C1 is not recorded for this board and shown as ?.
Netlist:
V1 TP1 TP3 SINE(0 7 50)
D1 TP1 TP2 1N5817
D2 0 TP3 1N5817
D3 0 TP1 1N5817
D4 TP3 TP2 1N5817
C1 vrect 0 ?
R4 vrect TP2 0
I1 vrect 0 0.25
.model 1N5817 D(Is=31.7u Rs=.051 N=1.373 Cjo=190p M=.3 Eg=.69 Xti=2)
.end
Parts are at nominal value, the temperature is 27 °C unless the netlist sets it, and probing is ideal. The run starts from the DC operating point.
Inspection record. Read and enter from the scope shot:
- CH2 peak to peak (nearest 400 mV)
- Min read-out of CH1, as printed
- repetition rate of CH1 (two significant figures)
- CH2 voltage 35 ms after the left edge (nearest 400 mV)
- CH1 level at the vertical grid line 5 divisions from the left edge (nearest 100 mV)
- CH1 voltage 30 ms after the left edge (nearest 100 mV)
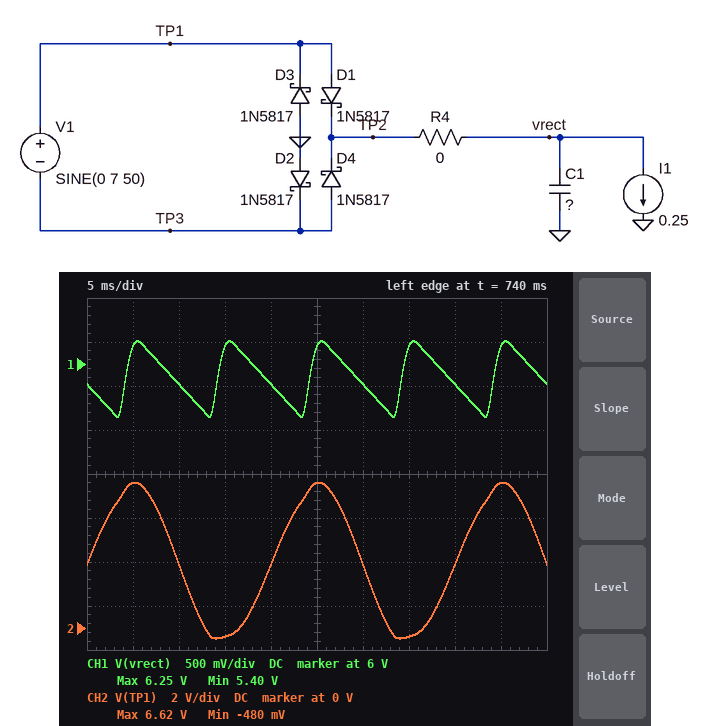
7.2 V
5.40 V
100 Hz
-400 mV
6.2 V
5.8 V
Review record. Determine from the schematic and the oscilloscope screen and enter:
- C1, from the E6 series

2.2 mF
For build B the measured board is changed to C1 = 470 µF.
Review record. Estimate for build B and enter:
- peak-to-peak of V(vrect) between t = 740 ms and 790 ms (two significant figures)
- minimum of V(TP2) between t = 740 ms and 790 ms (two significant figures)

3.2 V
3.1 V
